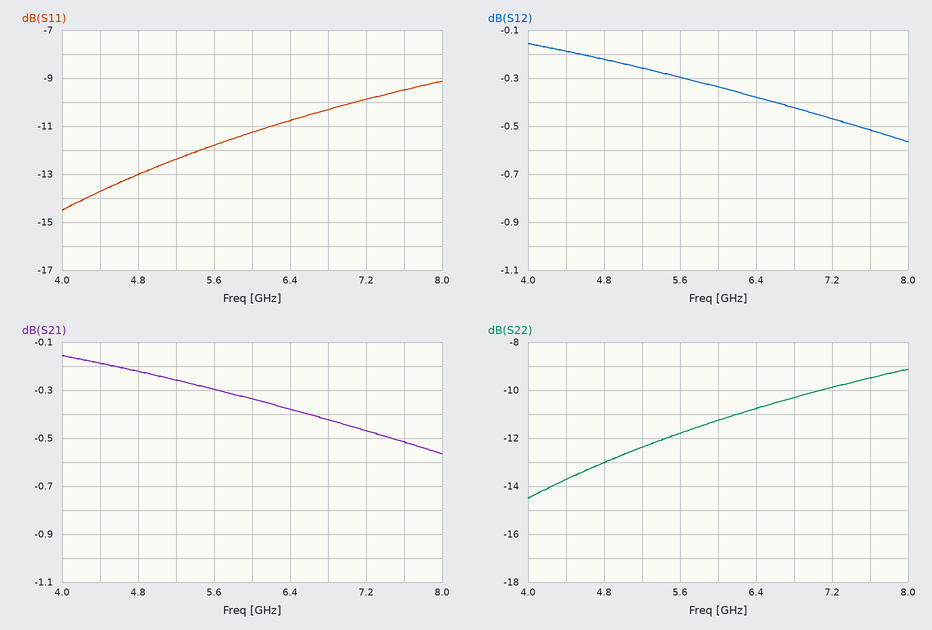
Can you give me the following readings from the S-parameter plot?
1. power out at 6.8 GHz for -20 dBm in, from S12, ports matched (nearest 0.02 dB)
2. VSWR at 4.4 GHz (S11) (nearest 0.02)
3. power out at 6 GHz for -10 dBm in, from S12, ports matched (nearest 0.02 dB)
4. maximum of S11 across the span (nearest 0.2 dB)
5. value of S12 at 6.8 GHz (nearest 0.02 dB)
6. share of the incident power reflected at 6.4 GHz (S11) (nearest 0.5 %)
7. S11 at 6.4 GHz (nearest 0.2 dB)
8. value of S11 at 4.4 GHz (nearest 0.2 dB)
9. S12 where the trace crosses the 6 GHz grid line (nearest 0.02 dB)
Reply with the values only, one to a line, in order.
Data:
-20.42 dBm
1.52
-10.34 dBm
-9.2 dB
-0.42 dB
8.5 %
-10.8 dB
-13.8 dB
-0.34 dB
